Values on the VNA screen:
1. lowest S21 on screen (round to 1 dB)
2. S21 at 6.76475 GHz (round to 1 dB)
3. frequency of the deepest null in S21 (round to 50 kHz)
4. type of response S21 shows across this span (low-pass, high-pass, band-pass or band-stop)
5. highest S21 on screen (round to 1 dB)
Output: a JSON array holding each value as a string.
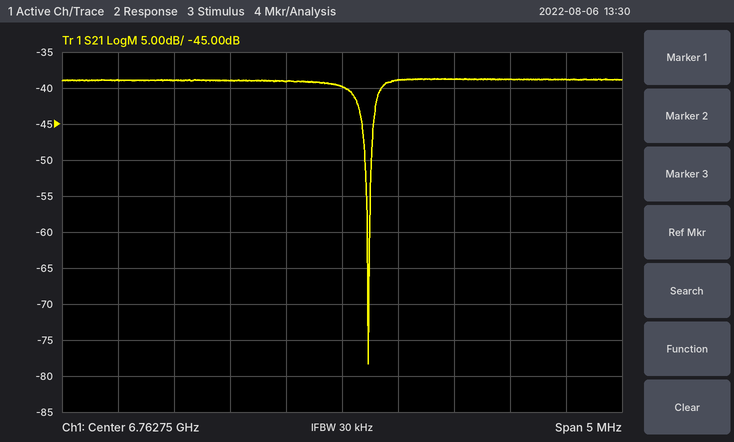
["-78 dB", "-39 dB", "6.76300 GHz", "band-stop", "-39 dB"]
